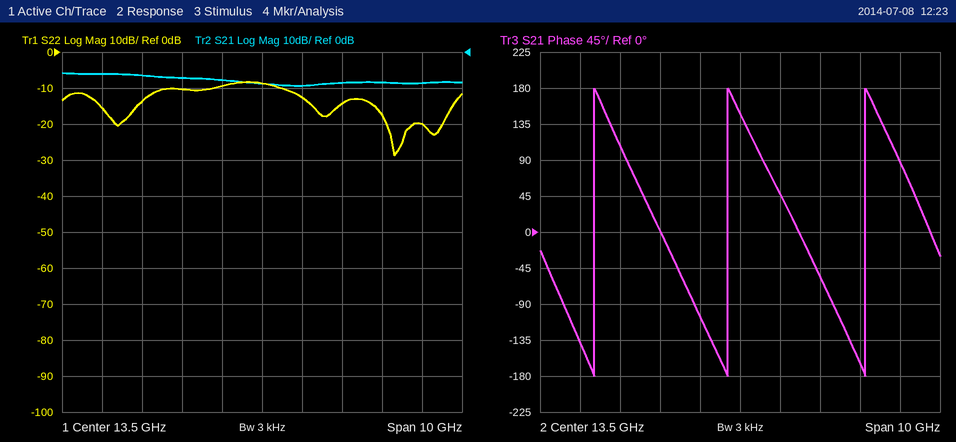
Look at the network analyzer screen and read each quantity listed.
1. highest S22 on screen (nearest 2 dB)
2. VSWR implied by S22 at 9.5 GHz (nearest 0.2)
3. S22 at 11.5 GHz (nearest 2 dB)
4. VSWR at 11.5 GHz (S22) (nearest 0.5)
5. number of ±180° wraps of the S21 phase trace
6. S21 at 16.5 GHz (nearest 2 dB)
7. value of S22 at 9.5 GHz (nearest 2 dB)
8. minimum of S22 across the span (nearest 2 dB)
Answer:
-8 dB
1.4
-10 dB
2.0
3
-8 dB
-16 dB
-28 dB
